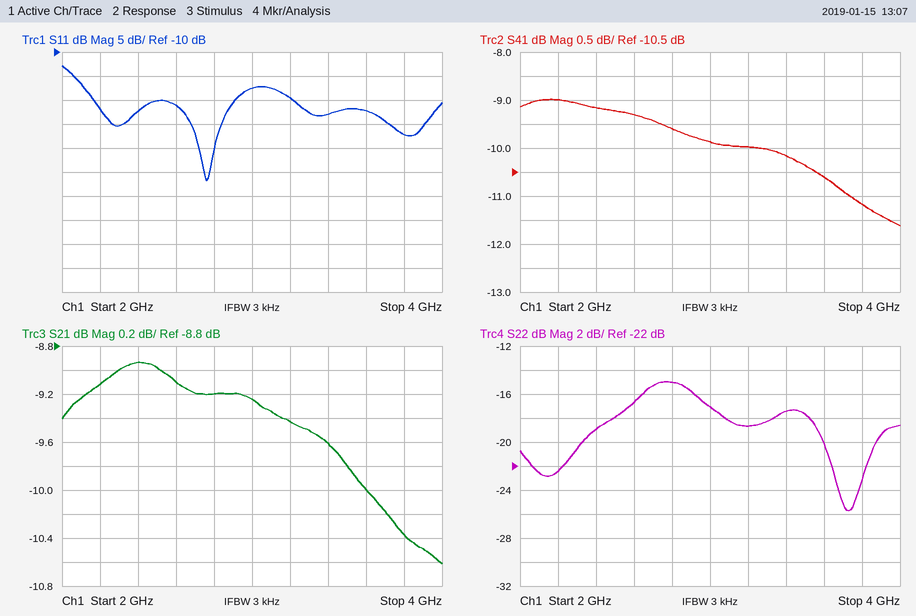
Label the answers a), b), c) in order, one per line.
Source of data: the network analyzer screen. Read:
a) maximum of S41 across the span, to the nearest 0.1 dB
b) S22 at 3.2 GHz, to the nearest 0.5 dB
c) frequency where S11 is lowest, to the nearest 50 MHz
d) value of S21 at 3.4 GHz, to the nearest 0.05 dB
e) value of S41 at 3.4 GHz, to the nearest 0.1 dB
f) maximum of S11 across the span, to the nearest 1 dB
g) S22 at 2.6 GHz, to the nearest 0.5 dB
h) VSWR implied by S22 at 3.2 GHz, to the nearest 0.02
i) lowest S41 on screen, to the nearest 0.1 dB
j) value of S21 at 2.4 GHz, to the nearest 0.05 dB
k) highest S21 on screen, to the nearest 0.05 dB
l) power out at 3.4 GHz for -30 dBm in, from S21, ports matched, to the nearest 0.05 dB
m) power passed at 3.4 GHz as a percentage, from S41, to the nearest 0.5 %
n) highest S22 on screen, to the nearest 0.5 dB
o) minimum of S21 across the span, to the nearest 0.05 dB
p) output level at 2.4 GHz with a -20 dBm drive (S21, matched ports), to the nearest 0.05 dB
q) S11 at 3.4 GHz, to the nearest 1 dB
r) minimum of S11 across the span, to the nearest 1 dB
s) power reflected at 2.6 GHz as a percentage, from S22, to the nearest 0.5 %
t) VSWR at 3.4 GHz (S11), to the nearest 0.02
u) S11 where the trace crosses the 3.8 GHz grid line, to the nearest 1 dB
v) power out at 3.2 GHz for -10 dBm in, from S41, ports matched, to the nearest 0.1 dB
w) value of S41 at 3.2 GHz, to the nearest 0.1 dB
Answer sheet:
a) -9.0 dB
b) -18.5 dB
c) 2.75 GHz
d) -9.60 dB
e) -10.2 dB
f) -13 dB
g) -16.5 dB
h) 1.26
i) -11.6 dB
j) -8.95 dB
k) -8.95 dB
l) -39.60 dBm
m) 9.5 %
n) -15.0 dB
o) -10.60 dB
p) -28.95 dBm
q) -23 dB
r) -37 dB
s) 2.0 %
t) 1.16
u) -27 dB
v) -20.0 dBm
w) -10.0 dB
